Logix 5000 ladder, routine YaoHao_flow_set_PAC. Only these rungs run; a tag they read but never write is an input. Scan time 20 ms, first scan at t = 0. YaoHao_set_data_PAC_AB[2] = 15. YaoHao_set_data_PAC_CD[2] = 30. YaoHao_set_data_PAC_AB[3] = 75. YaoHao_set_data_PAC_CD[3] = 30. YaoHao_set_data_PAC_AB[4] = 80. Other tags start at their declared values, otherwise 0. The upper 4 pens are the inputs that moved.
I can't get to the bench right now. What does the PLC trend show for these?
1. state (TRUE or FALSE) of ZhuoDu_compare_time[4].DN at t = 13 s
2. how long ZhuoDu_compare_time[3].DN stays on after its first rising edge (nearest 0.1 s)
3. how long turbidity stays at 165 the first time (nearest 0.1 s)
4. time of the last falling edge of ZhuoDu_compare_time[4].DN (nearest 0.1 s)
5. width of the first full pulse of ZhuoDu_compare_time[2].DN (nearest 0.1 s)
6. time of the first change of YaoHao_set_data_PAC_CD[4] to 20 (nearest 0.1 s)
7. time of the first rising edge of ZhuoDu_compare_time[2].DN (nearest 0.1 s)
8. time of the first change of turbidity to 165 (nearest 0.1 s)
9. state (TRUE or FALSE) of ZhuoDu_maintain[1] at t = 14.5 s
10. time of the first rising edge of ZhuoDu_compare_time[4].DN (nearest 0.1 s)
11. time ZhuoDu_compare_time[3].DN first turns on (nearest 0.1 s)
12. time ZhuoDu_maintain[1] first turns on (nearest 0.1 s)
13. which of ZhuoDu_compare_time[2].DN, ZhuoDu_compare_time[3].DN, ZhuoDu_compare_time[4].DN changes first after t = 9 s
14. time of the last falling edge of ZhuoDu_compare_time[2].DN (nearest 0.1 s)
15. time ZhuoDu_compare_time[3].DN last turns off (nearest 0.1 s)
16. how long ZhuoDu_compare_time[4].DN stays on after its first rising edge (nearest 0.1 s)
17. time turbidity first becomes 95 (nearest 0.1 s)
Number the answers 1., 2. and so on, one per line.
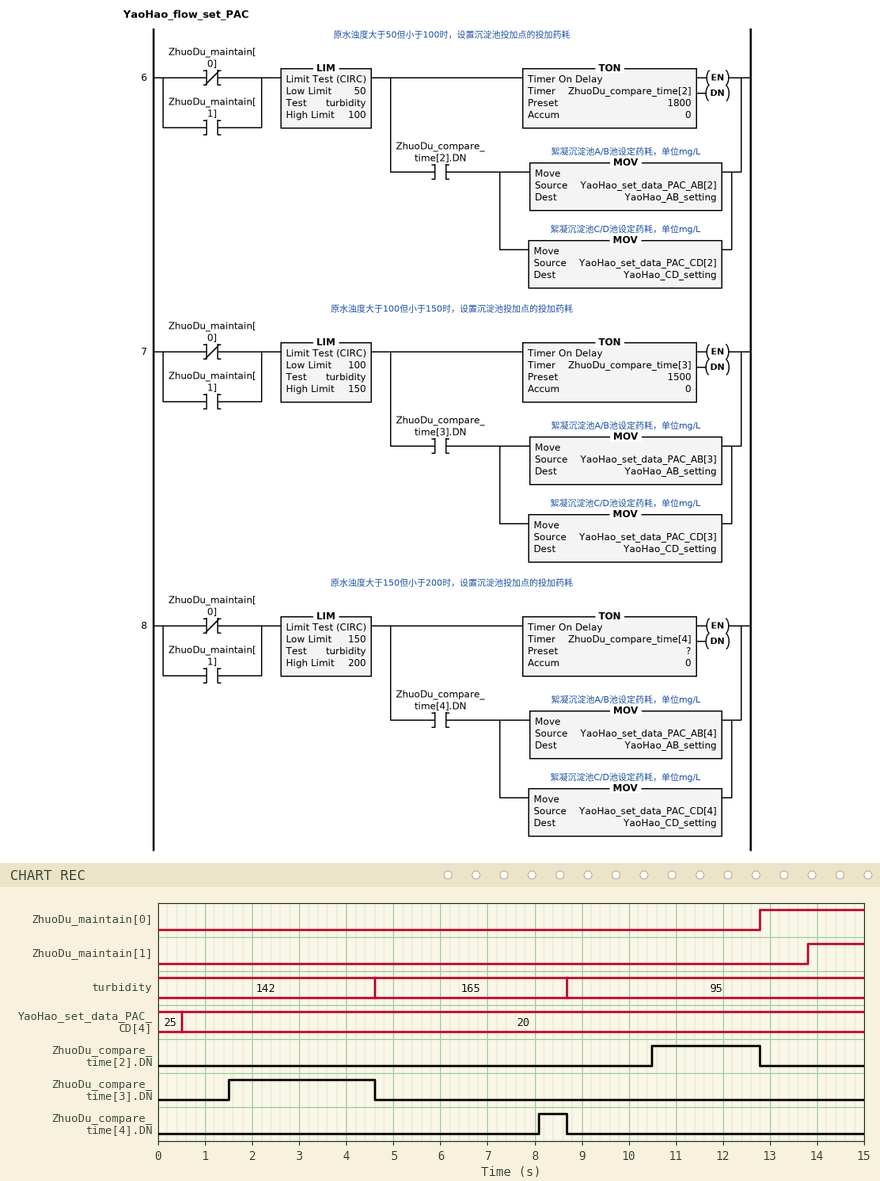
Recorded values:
1. FALSE
2. 3.1 s
3. 4.1 s
4. 8.7 s
5. 2.3 s
6. 0.5 s
7. 10.5 s
8. 4.6 s
9. TRUE
10. 8.1 s
11. 1.5 s
12. 13.8 s
13. ZhuoDu_compare_time[2].DN
14. 12.8 s
15. 4.6 s
16. 0.6 s
17. 8.7 s
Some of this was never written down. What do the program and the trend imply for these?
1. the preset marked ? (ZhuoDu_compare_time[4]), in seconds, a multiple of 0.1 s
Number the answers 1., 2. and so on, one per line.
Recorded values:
1. 3.5 s
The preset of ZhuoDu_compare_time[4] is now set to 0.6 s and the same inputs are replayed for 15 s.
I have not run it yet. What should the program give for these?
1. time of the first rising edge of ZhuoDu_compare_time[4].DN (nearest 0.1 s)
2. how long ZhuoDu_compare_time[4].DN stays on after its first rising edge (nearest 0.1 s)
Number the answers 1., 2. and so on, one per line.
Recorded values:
1. 5.2 s
2. 3.5 s
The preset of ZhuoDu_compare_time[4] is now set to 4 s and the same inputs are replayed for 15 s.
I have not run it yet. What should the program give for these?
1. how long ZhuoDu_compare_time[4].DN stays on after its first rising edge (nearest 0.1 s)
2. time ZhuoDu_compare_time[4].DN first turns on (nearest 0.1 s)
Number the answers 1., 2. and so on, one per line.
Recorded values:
1. 0.1 s
2. 8.6 s
